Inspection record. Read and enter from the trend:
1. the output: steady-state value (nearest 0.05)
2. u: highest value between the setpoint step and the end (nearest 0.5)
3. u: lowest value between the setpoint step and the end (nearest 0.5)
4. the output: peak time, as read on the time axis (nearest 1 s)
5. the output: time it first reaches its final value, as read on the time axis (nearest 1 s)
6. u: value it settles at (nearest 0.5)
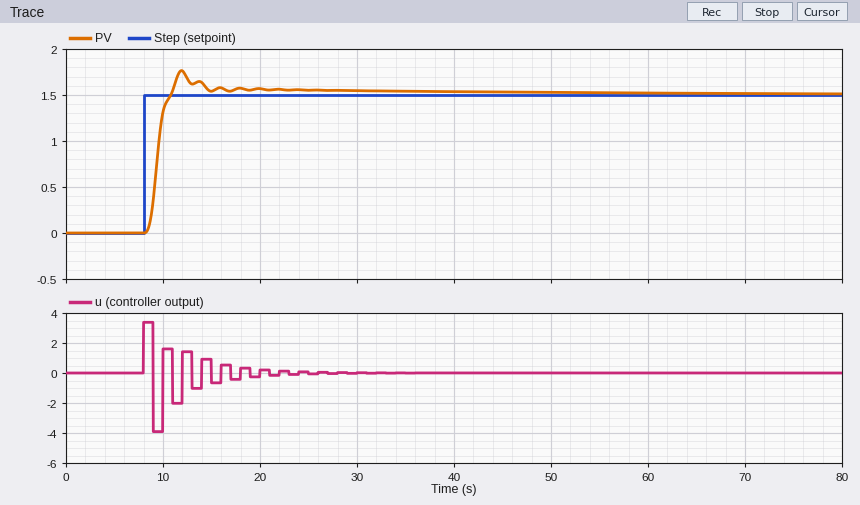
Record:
1.50
3.5
-4.0
12 s
11 s
0.0
